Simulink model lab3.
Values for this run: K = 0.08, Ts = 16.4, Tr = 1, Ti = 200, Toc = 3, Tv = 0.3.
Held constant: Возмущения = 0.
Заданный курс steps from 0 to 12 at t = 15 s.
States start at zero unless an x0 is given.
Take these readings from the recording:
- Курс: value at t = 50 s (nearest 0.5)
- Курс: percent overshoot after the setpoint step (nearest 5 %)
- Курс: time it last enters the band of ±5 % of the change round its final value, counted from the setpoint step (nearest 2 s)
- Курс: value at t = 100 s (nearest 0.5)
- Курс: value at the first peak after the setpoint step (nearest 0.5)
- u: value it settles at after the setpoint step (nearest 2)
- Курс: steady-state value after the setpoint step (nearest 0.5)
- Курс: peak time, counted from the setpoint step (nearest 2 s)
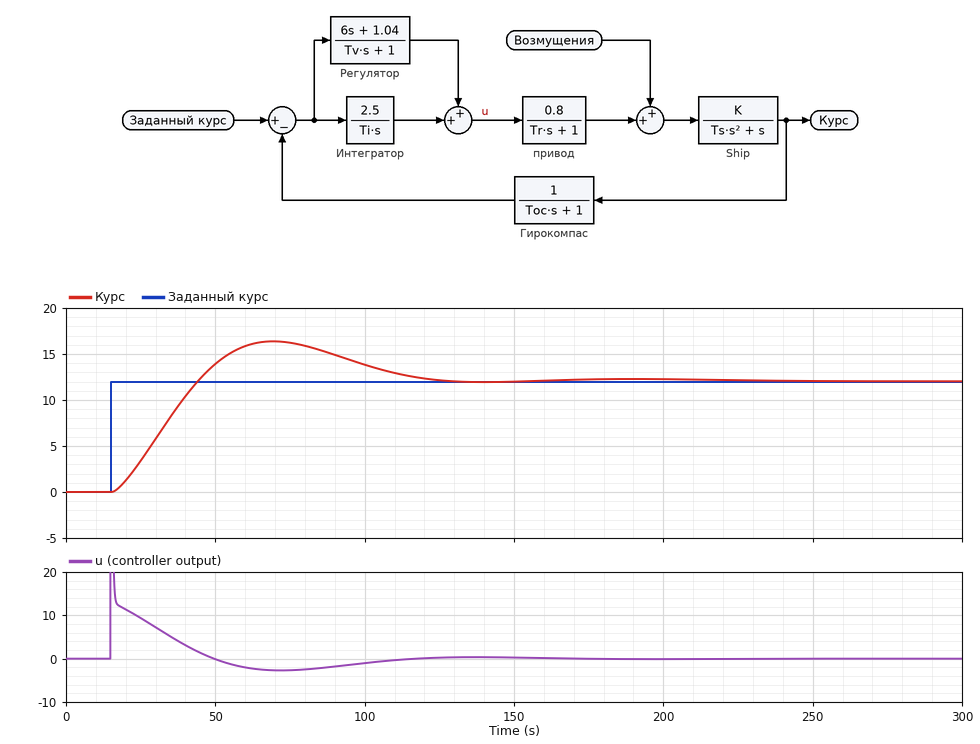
14.0
35 %
100 s
14.0
16.5
0
12.0
54 s
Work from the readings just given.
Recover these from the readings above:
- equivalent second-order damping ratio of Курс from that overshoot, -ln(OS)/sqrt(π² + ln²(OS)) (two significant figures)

0.32
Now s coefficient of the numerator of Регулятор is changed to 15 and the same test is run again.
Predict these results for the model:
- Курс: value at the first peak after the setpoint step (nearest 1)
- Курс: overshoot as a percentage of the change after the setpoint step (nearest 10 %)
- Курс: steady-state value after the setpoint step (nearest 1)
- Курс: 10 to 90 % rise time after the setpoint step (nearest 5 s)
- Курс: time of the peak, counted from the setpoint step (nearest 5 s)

14
20 %
12
20 s
60 s
